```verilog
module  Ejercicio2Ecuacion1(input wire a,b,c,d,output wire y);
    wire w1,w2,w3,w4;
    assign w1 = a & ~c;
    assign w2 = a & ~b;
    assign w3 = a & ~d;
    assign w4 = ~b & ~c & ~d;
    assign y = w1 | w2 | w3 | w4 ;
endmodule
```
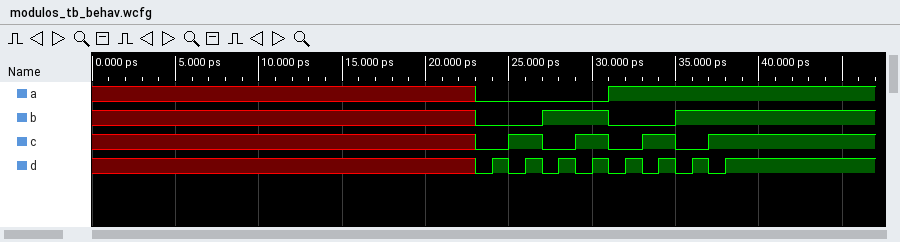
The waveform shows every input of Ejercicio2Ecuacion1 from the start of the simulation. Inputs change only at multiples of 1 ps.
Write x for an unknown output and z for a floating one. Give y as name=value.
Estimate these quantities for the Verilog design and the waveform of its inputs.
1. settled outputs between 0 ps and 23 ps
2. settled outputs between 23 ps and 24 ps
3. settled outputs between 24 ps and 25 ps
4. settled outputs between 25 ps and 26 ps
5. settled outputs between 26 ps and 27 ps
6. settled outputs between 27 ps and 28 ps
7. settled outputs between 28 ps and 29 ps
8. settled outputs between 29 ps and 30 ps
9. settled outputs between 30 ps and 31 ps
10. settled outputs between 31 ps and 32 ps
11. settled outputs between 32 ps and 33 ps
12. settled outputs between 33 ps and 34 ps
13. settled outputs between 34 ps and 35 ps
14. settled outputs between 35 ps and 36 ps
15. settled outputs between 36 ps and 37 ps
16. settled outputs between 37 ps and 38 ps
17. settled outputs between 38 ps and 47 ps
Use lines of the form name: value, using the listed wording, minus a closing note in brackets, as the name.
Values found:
settled outputs between 0 ps and 23 ps: y=x
settled outputs between 23 ps and 24 ps: y=1
settled outputs between 24 ps and 25 ps: y=0
settled outputs between 25 ps and 26 ps: y=0
settled outputs between 26 ps and 27 ps: y=0
settled outputs between 27 ps and 28 ps: y=0
settled outputs between 28 ps and 29 ps: y=0
settled outputs between 29 ps and 30 ps: y=0
settled outputs between 30 ps and 31 ps: y=0
settled outputs between 31 ps and 32 ps: y=1
settled outputs between 32 ps and 33 ps: y=1
settled outputs between 33 ps and 34 ps: y=1
settled outputs between 34 ps and 35 ps: y=1
settled outputs between 35 ps and 36 ps: y=1
settled outputs between 36 ps and 37 ps: y=1
settled outputs between 37 ps and 38 ps: y=1
settled outputs between 38 ps and 47 ps: y=0
